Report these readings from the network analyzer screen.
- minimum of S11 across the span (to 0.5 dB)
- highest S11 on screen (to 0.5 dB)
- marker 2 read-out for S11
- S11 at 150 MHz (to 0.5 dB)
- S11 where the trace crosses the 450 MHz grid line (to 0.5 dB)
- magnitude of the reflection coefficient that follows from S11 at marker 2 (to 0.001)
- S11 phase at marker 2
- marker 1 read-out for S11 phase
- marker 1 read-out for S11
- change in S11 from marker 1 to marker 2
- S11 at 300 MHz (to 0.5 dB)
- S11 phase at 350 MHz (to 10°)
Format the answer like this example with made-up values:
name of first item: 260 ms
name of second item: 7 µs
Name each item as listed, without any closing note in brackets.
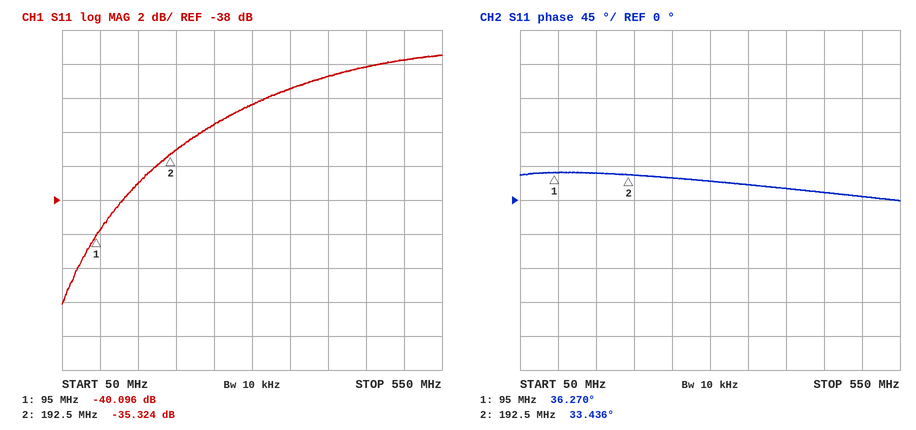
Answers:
minimum of S11 across the span: -44.0 dB
highest S11 on screen: -29.5 dB
marker 2 read-out for S11: -35.324 dB
S11 at 150 MHz: -37.0 dB
S11 where the trace crosses the 450 MHz grid line: -30.0 dB
magnitude of the reflection coefficient that follows from S11 at marker 2: 0.017
S11 phase at marker 2: 33.436°
marker 1 read-out for S11 phase: 36.270°
marker 1 read-out for S11: -40.096 dB
change in S11 from marker 1 to marker 2: 4.772 dB
S11 at 300 MHz: -32.5 dB
S11 phase at 350 MHz: 20°
